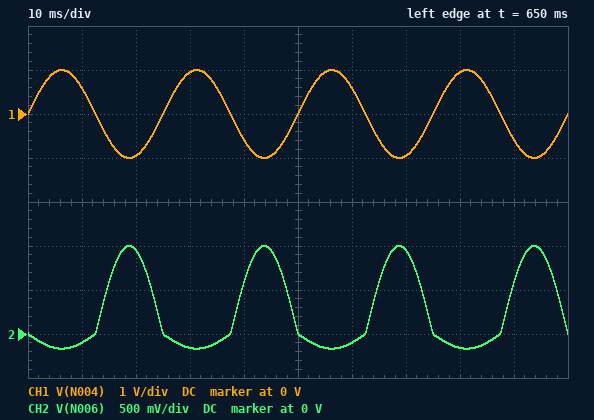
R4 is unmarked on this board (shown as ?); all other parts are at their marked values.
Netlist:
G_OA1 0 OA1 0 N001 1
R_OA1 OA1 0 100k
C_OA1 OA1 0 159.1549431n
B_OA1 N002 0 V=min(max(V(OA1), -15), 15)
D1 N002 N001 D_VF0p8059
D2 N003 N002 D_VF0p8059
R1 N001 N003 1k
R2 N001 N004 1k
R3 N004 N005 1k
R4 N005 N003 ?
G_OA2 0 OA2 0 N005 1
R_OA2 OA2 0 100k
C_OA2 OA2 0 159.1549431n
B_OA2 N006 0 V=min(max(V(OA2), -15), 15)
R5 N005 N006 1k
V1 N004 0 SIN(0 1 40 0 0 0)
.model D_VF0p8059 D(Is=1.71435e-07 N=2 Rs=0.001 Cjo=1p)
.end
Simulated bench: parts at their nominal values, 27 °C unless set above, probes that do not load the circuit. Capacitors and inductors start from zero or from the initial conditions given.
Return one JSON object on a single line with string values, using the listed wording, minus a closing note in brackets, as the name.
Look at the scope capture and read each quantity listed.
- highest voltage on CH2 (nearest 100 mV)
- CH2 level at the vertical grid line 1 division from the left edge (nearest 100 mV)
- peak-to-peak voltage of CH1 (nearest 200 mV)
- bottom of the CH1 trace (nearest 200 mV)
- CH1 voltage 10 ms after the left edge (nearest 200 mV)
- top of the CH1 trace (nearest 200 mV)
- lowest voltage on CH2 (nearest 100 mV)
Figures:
{"highest voltage on CH2": "1.0 V", "CH2 level at the vertical grid line 1 division from the left edge": "-100 mV", "peak-to-peak voltage of CH1": "2.0 V", "bottom of the CH1 trace": "-1.0 V", "CH1 voltage 10 ms after the left edge": "600 mV", "top of the CH1 trace": "1.0 V", "lowest voltage on CH2": "-200 mV"}
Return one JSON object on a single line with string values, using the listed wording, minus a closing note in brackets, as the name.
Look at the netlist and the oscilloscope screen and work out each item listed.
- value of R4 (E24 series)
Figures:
{"value of R4": "1.2 kΩ"}
